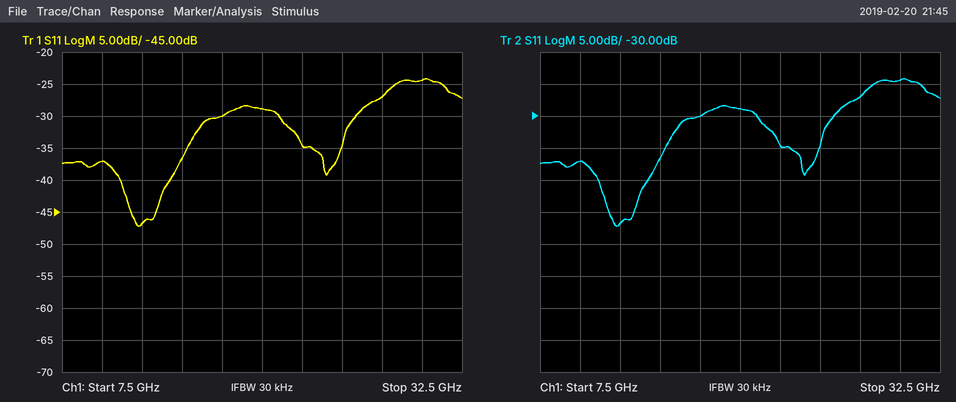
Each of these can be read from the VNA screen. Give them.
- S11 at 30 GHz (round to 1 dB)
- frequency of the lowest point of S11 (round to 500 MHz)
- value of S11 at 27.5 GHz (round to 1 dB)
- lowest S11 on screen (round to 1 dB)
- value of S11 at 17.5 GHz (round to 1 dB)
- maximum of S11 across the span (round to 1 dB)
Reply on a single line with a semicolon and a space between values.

-24 dB; 12.5 GHz; -27 dB; -47 dB; -30 dB; -24 dB
